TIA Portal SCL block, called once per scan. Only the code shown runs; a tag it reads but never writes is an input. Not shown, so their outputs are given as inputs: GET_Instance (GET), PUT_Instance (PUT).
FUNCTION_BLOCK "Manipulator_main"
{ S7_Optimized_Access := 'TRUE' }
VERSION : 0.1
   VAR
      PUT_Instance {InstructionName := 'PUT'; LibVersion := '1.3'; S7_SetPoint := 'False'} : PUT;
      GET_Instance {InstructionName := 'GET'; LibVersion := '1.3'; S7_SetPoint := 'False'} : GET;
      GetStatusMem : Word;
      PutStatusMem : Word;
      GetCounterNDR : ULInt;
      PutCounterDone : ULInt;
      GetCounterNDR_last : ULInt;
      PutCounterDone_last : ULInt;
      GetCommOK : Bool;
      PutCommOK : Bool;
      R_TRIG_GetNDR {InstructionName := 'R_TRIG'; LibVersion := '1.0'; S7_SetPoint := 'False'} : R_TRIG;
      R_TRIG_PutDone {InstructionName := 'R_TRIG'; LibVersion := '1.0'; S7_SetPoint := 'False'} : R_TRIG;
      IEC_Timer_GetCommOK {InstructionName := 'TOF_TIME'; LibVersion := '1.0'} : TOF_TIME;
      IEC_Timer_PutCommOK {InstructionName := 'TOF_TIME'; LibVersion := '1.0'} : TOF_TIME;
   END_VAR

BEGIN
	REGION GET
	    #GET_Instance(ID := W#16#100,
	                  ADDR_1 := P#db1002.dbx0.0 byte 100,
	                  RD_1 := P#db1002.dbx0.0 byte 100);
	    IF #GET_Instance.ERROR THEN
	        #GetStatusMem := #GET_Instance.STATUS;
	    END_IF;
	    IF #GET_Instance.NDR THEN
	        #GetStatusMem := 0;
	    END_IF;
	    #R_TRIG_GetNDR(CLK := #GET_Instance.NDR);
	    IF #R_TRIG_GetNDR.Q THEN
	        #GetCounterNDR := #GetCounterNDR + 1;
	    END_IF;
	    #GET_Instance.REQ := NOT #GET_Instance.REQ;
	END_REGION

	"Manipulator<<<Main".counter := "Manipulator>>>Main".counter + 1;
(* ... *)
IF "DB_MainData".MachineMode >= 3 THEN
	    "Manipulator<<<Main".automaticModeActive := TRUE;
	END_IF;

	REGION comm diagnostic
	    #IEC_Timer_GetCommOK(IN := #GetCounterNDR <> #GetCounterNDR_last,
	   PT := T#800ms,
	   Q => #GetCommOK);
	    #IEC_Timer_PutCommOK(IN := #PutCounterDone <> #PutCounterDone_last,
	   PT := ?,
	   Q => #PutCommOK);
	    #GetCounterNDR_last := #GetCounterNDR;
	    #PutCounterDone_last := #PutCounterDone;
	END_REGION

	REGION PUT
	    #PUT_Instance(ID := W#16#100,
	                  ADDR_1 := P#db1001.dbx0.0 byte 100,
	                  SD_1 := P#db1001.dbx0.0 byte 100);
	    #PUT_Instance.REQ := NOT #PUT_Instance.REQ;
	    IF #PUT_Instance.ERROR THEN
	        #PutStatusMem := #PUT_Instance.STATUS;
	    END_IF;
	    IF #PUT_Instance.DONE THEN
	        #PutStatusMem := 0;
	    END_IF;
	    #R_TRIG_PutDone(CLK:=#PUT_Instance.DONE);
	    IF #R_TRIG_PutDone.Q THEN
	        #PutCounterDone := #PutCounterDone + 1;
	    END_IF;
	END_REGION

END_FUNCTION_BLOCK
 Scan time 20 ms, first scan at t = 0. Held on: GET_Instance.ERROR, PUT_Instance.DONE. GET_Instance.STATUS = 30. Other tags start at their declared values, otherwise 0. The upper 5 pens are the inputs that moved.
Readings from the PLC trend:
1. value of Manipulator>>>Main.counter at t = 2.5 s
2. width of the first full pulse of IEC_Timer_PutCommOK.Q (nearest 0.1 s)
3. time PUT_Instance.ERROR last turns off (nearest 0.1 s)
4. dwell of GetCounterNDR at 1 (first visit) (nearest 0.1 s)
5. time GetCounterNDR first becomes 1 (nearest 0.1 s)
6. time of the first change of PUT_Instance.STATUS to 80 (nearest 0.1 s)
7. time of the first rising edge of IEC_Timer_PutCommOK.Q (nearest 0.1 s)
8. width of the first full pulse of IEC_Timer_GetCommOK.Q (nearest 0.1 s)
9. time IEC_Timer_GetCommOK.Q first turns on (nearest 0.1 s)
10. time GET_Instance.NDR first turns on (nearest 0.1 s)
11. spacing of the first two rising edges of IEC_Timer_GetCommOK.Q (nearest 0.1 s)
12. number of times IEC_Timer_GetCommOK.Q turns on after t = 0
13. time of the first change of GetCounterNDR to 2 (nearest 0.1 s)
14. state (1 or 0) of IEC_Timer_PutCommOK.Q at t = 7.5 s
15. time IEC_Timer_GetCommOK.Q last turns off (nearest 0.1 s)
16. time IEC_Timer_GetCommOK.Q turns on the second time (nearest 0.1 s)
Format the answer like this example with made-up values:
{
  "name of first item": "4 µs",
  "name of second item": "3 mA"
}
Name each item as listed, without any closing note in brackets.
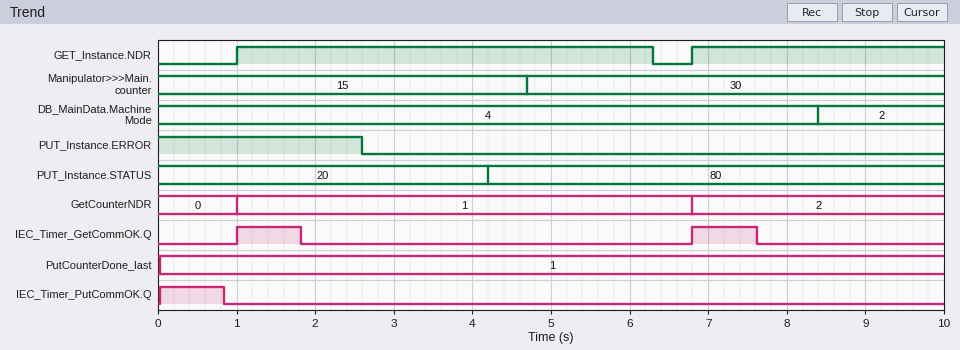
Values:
{
  "value of Manipulator>>>Main.counter at t = 2.5 s": "15",
  "width of the first full pulse of IEC_Timer_PutCommOK.Q": "0.8 s",
  "time PUT_Instance.ERROR last turns off": "2.6 s",
  "dwell of GetCounterNDR at 1 (first visit)": "5.8 s",
  "time GetCounterNDR first becomes 1": "1.0 s",
  "time of the first change of PUT_Instance.STATUS to 80": "4.2 s",
  "time of the first rising edge of IEC_Timer_PutCommOK.Q": "0.0 s",
  "width of the first full pulse of IEC_Timer_GetCommOK.Q": "0.8 s",
  "time IEC_Timer_GetCommOK.Q first turns on": "1.0 s",
  "time GET_Instance.NDR first turns on": "1.0 s",
  "spacing of the first two rising edges of IEC_Timer_GetCommOK.Q": "5.8 s",
  "number of times IEC_Timer_GetCommOK.Q turns on after t = 0": "2",
  "time of the first change of GetCounterNDR to 2": "6.8 s",
  "state (1 or 0) of IEC_Timer_PutCommOK.Q at t = 7.5 s": "0",
  "time IEC_Timer_GetCommOK.Q last turns off": "7.6 s",
  "time IEC_Timer_GetCommOK.Q turns on the second time": "6.8 s"
}
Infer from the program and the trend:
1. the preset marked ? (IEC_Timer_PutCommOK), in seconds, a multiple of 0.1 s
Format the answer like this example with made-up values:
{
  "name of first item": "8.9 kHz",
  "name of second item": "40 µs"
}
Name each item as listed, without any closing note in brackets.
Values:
{
  "the preset marked ? (IEC_Timer_PutCommOK), in seconds, a multiple of 0.1 s": "0.8 s"
}
